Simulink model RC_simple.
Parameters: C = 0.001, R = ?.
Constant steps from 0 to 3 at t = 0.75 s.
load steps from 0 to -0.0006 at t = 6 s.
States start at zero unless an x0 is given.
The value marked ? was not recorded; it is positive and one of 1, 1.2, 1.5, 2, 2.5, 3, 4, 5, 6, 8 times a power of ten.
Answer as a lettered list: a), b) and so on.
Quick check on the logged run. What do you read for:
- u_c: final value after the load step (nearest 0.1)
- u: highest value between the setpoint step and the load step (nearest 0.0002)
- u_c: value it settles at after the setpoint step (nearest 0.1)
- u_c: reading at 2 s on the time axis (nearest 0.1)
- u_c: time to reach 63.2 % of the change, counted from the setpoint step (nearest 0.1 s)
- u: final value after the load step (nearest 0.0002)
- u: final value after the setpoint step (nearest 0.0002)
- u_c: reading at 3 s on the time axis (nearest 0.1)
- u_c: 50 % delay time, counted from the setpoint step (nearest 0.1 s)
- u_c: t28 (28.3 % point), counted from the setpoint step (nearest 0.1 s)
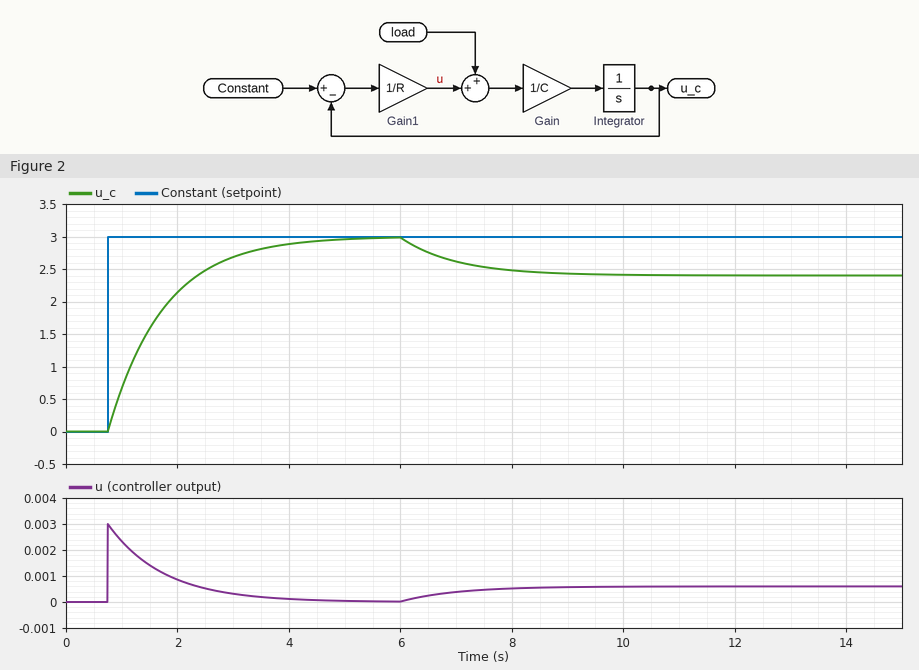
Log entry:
a) 2.4
b) 0.0030
c) 3.0
d) 2.1
e) 1.0 s
f) 0.0006
g) 0.0000
h) 2.7
i) 0.7 s
j) 0.3 s
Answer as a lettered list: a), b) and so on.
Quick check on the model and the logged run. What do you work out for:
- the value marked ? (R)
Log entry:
a) 1000
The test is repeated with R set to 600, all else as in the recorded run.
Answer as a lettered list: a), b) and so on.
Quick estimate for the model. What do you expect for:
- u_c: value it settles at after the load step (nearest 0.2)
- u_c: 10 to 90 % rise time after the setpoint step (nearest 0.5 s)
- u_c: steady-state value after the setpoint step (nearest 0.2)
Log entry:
a) 2.6
b) 1.5 s
c) 3.0
